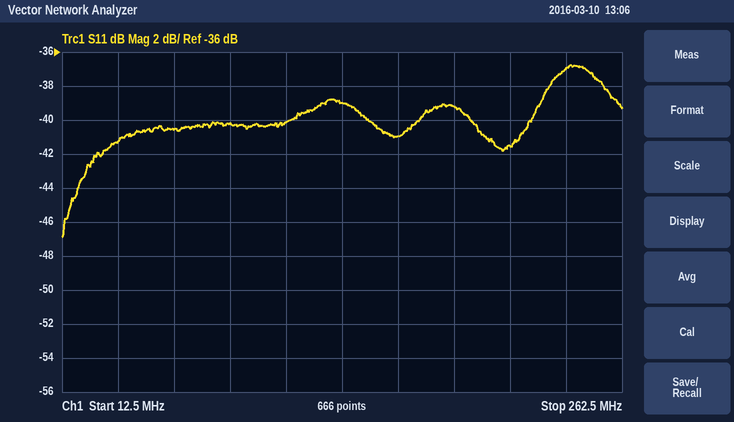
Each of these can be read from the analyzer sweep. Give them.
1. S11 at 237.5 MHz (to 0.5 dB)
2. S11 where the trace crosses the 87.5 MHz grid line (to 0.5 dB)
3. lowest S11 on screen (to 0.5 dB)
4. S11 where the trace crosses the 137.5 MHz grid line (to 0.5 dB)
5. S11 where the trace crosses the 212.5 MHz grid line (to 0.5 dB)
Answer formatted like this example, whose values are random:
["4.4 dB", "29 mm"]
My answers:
["-37.0 dB", "-40.0 dB", "-47.0 dB", "-39.0 dB", "-41.5 dB"]
